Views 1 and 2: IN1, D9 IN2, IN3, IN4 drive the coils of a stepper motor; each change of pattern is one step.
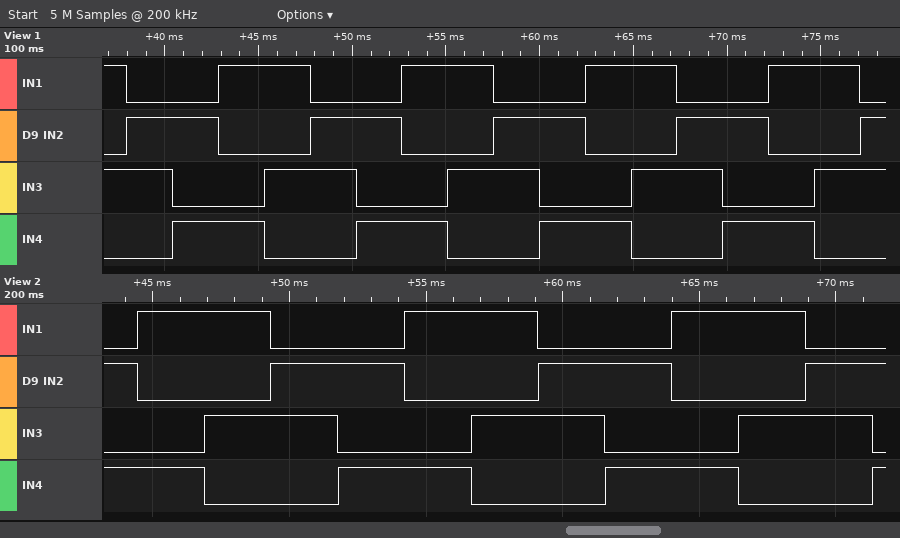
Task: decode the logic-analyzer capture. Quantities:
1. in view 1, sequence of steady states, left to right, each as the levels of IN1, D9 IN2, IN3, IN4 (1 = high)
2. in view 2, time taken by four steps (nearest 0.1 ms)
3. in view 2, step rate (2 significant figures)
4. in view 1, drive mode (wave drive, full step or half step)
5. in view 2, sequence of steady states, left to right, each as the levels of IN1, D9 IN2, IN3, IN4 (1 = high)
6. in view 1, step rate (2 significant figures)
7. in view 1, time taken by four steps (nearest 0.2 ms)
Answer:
1010 0110 0101 1001 1010 0110 0101 1001 1010 0110 0101 1001 1010 0110 0101 1001 1010 0110
9.8 ms
410 steps/s
full step
0101 1001 1010 0110 0101 1001 1010 0110 0101 1001 1010 0110 0101
410 steps/s
9.8 ms
